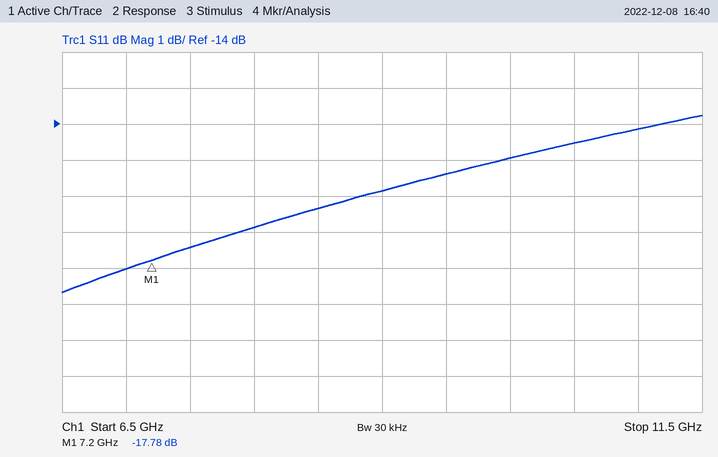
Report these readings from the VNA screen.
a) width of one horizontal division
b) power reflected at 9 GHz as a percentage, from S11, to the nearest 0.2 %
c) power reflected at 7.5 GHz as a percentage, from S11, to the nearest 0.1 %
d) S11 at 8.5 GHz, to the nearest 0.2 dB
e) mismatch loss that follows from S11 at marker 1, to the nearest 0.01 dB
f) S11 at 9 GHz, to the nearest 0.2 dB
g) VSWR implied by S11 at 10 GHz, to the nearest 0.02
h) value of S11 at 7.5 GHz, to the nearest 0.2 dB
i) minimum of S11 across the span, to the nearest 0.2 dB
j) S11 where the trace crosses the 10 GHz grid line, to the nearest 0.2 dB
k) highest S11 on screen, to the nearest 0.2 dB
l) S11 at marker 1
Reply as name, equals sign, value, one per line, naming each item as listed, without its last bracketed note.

width of one horizontal division = 500 MHz
power reflected at 9 GHz as a percentage, from S11, to the nearest 0.2 % = 2.6 %
power reflected at 7.5 GHz as a percentage, from S11, to the nearest 0.1 % = 1.8 %
S11 at 8.5 GHz, to the nearest 0.2 dB = -16.4 dB
mismatch loss that follows from S11 at marker 1, to the nearest 0.01 dB = 0.07 dB
S11 at 9 GHz, to the nearest 0.2 dB = -15.8 dB
VSWR implied by S11 at 10 GHz, to the nearest 0.02 = 1.44
value of S11 at 7.5 GHz, to the nearest 0.2 dB = -17.4 dB
minimum of S11 across the span, to the nearest 0.2 dB = -18.6 dB
S11 where the trace crosses the 10 GHz grid line, to the nearest 0.2 dB = -15.0 dB
highest S11 on screen, to the nearest 0.2 dB = -13.8 dB
S11 at marker 1 = -17.78 dB
